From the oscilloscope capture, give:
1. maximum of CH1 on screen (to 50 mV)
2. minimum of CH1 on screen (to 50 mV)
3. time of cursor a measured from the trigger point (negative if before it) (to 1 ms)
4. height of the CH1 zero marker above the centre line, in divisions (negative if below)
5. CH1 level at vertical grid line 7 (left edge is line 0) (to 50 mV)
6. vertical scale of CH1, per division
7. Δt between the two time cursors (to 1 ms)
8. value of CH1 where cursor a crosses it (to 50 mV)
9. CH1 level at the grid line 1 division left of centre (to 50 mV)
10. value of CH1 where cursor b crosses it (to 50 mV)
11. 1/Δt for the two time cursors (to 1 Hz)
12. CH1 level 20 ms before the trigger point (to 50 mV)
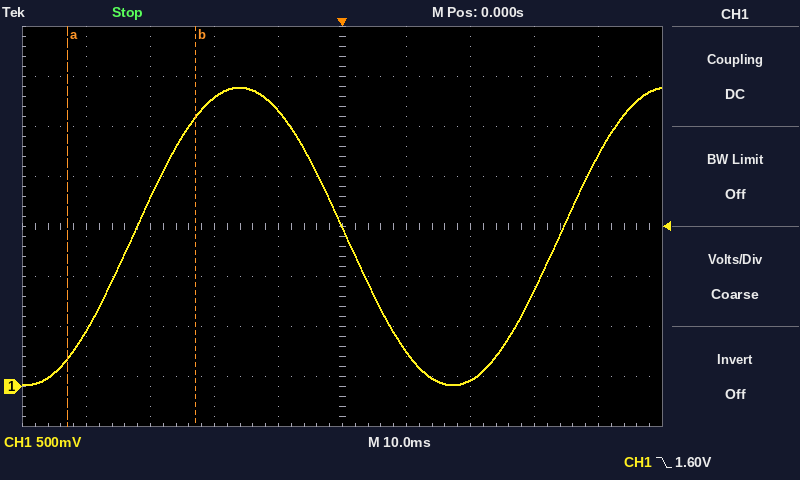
3.00 V
0 mV
-43 ms
-3.2 div
50 mV
500 mV
20 ms
300 mV
2.75 V
2.70 V
50 Hz
2.90 V
